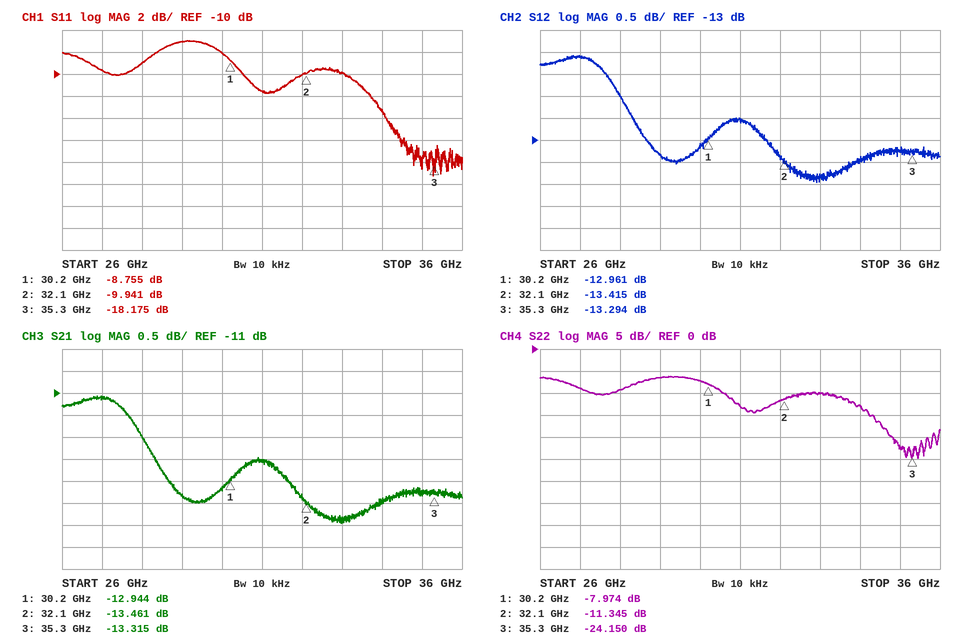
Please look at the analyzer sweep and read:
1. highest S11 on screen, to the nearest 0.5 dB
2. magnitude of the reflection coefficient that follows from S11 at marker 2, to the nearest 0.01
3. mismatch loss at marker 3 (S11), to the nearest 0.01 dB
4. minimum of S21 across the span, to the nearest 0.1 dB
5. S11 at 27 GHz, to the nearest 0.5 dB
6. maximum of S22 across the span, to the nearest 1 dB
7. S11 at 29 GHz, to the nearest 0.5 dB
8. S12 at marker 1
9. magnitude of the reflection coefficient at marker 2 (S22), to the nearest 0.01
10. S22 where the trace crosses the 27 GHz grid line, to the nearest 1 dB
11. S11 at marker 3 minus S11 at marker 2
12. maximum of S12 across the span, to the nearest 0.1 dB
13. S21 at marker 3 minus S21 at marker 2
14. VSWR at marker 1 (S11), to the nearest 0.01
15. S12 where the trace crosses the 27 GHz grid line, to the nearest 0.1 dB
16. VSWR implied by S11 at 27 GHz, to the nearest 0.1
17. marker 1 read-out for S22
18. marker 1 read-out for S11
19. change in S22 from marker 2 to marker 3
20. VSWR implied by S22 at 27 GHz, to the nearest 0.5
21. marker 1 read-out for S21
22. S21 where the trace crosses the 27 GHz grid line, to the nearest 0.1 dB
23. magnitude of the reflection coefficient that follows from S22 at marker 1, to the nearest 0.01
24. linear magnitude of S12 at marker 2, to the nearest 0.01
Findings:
-7.0 dB
0.32
0.07 dB
-14.0 dB
-9.5 dB
-6 dB
-7.0 dB
-12.961 dB
0.27
-9 dB
-8.234 dB
-11.1 dB
0.146 dB
2.15
-11.1 dB
2.0
-7.974 dB
-8.755 dB
-12.805 dB
2.0
-12.944 dB
-11.1 dB
0.40
0.21
